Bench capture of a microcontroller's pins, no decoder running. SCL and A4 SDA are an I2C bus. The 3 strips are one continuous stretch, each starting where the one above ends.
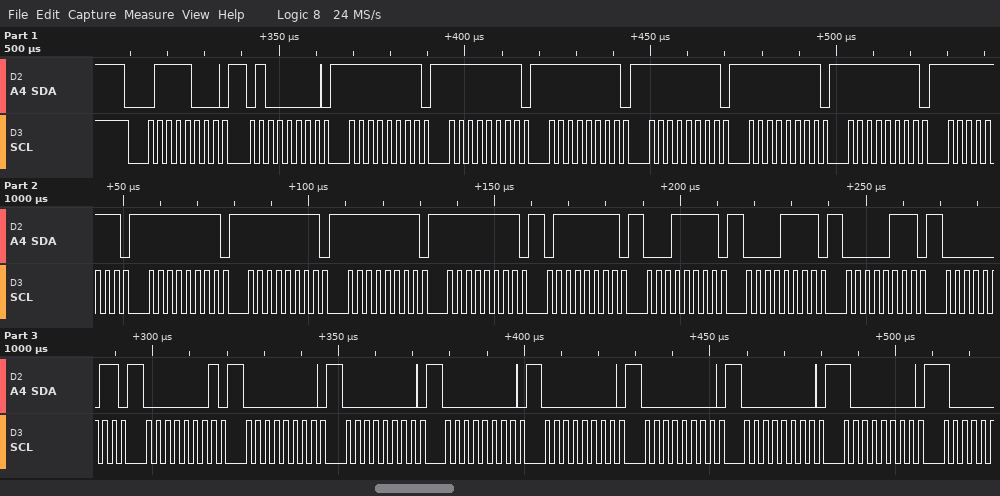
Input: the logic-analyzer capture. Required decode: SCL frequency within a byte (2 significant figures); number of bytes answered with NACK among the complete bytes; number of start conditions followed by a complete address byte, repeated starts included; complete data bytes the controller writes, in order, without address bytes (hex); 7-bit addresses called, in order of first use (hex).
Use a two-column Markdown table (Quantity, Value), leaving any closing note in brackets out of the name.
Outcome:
| Quantity | Value |
|---|---|
| SCL frequency within a byte | 400 kHz |
| number of bytes answered with NACK among the complete bytes | 0 |
| number of start conditions followed by a complete address byte, repeated starts included | 1 |
| complete data bytes the controller writes, in order, without address bytes | 40 FF FF FF FF FF FF FF FF FF FF FF 7F 1F 0F 07 03 01 00 00 00 00 00 00 80 |
| 7-bit addresses called, in order of first use | 0x3C |
